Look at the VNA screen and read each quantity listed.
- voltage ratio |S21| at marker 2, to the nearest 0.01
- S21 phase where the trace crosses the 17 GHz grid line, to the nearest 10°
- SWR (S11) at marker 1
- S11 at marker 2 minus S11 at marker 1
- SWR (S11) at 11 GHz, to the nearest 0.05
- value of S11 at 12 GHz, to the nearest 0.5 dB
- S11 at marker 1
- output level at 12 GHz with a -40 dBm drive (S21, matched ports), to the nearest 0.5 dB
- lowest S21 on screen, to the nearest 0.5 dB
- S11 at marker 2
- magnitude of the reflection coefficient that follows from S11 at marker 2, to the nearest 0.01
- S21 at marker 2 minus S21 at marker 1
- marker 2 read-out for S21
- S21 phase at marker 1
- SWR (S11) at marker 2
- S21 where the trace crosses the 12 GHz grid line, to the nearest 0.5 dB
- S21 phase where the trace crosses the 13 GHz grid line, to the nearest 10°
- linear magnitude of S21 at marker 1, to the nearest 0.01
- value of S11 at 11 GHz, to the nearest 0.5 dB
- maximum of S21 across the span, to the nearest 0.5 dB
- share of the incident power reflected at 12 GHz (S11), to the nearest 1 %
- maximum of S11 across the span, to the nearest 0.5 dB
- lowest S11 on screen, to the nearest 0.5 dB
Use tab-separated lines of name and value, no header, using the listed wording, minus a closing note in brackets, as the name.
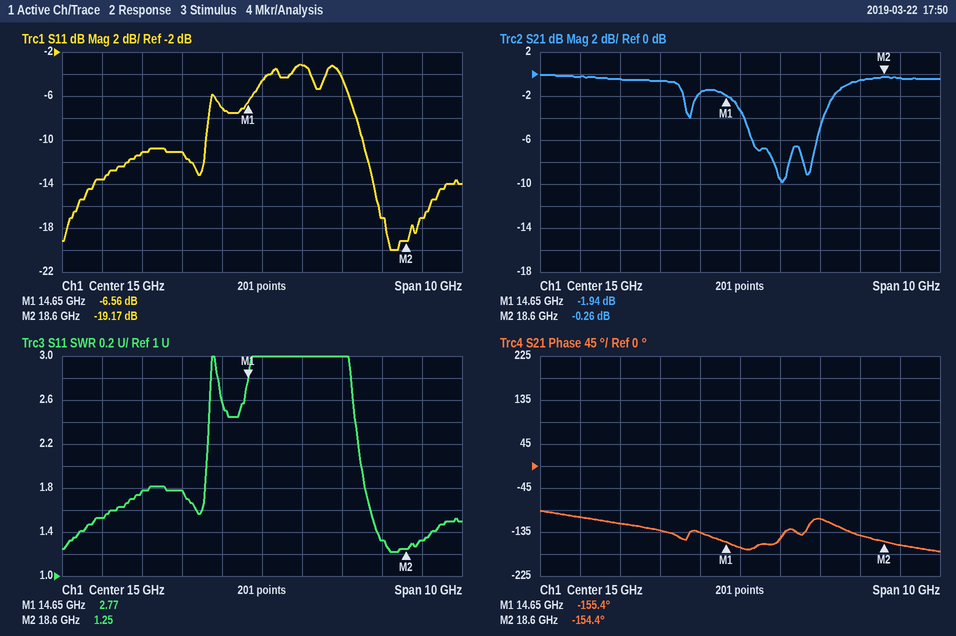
voltage ratio |S21| at marker 2, to the nearest 0.01	0.97
S21 phase where the trace crosses the 17 GHz grid line, to the nearest 10°	-110°
SWR (S11) at marker 1	2.77
S11 at marker 2 minus S11 at marker 1	-12.61 dB
SWR (S11) at 11 GHz, to the nearest 0.05	1.55
value of S11 at 12 GHz, to the nearest 0.5 dB	-11.0 dB
S11 at marker 1	-6.56 dB
output level at 12 GHz with a -40 dBm drive (S21, matched ports), to the nearest 0.5 dB	-40.5 dBm
lowest S21 on screen, to the nearest 0.5 dB	-10.0 dB
S11 at marker 2	-19.17 dB
magnitude of the reflection coefficient that follows from S11 at marker 2, to the nearest 0.01	0.11
S21 at marker 2 minus S21 at marker 1	1.68 dB
marker 2 read-out for S21	-0.26 dB
S21 phase at marker 1	-155.4°
SWR (S11) at marker 2	1.25
S21 where the trace crosses the 12 GHz grid line, to the nearest 0.5 dB	-0.5 dB
S21 phase where the trace crosses the 13 GHz grid line, to the nearest 10°	-130°
linear magnitude of S21 at marker 1, to the nearest 0.01	0.80
value of S11 at 11 GHz, to the nearest 0.5 dB	-13.5 dB
maximum of S21 across the span, to the nearest 0.5 dB	0.0 dB
share of the incident power reflected at 12 GHz (S11), to the nearest 1 %	8 %
maximum of S11 across the span, to the nearest 0.5 dB	-3.0 dB
lowest S11 on screen, to the nearest 0.5 dB	-20.0 dB
